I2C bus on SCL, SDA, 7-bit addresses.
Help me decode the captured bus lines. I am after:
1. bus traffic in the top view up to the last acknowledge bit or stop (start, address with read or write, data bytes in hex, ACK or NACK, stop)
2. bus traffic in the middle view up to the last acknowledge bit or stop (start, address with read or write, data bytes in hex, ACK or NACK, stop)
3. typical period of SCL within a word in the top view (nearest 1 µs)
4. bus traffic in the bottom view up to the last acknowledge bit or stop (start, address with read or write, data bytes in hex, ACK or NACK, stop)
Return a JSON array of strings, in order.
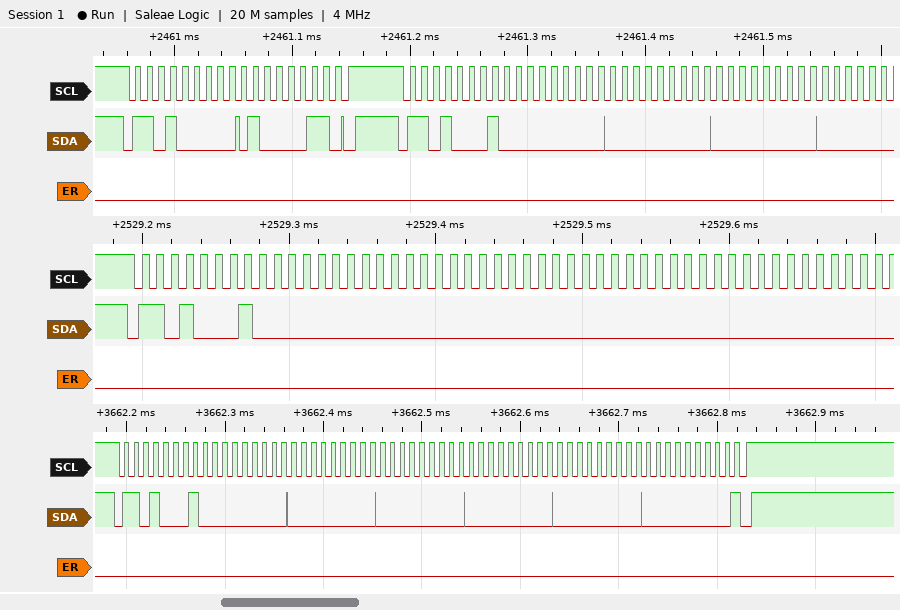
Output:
["start, address 68 write ACK, 43 ACK, stop, start, address 68 read ACK, 00 ACK, 00 ACK, 00 ACK", "start, address 68 read ACK, 00 ACK, 00 ACK, 00 ACK, 00 ACK", "10 µs", "start, address 68 read ACK, 00 ACK, 00 ACK, 00 ACK, 00 ACK, 00 ACK, 00 NACK, stop"]
